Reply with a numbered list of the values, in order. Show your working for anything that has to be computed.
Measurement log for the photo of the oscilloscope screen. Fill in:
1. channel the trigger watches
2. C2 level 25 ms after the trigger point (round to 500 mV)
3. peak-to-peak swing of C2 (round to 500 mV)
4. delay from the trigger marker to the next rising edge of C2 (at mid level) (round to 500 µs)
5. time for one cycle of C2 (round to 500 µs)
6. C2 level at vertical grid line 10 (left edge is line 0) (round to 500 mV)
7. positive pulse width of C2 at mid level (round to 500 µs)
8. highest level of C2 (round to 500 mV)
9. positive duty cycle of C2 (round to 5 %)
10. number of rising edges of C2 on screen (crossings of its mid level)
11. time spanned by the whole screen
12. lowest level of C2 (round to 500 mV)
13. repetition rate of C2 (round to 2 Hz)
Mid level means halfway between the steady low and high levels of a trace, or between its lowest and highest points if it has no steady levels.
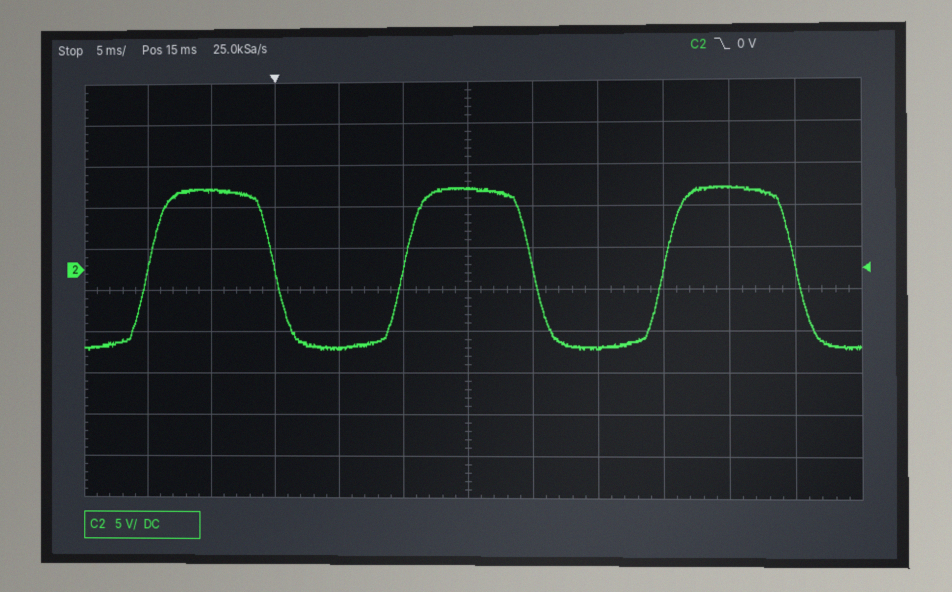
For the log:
1. C2
2. -9.5 V
3. 10.0 V − (-9.5 V) = 19.5 V
4. 10.0 ms
5. 20.0 ms
6. 9.5 V
7. 10.0 ms
8. 10.0 V
9. 10.0 ms / 20.0 ms ≈ 50 %
10. 3
11. 60 ms
12. -9.5 V
13. 1 / 20.0 ms ≈ 50 Hz
